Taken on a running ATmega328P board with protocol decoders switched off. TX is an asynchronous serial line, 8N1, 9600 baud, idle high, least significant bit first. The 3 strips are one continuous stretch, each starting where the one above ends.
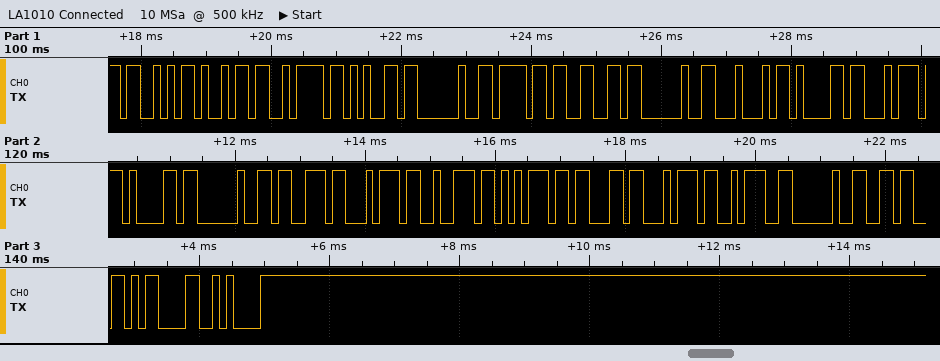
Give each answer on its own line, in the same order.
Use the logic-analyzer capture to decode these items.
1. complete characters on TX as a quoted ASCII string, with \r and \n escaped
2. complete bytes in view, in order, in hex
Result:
"Size of Data struct: 6\r\n"
53 69 7A 65 20 6F 66 20 44 61 74 61 20 73 74 72 75 63 74 3A 20 36 0D 0A
